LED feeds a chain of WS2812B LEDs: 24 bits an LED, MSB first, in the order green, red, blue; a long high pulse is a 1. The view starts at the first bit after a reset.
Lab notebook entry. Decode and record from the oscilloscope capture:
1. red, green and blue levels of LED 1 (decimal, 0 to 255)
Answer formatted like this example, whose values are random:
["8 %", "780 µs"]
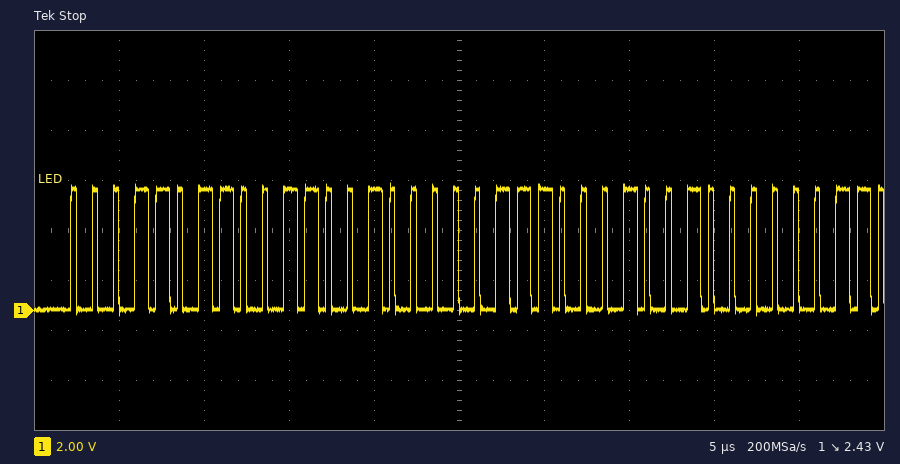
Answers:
["50, 27, 14"]
